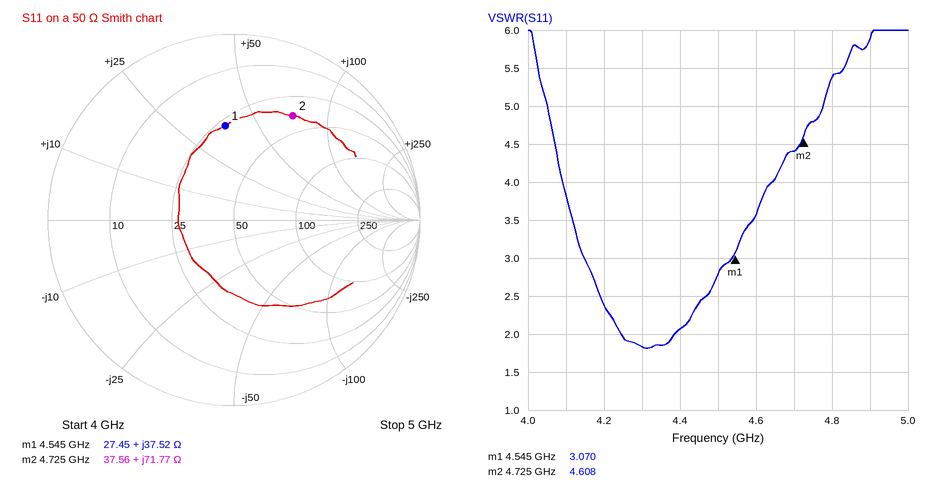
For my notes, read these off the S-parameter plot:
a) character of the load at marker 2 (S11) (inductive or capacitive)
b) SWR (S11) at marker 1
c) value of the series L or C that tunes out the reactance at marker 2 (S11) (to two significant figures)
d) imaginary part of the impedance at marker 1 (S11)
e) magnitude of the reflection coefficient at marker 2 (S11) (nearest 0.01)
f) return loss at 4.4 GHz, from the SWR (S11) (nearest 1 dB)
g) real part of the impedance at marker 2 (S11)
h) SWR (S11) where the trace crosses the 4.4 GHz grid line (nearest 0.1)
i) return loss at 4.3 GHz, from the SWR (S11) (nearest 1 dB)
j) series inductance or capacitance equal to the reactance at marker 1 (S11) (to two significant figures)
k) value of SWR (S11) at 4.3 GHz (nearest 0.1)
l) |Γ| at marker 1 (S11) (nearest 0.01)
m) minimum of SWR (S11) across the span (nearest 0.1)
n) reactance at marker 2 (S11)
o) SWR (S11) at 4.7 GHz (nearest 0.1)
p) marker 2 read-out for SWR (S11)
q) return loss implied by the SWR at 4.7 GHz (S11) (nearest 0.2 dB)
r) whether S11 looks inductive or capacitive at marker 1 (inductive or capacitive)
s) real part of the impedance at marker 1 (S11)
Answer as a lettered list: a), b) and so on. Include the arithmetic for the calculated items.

a) inductive
b) 3.070
c) C = 1/(2π × 4.725 GHz × 71.77 Ω) ≈ 469 fF, so 470 fF to two significant figures
d) +37.52 Ω
e) 0.64
f) −20 log10((2.1 − 1)/(2.1 + 1)) ≈ 9 dB
g) 37.56 Ω
h) 2.1
i) −20 log10((1.8 − 1)/(1.8 + 1)) ≈ 11 dB
j) L = 37.52 Ω/(2π × 4.545 GHz) ≈ 1.3 nH
k) 1.8
l) 0.51
m) 1.8
n) +71.77 Ω
o) 4.4
p) 4.608
q) −20 log10((4.4 − 1)/(4.4 + 1)) ≈ 4.0 dB
r) inductive
s) 27.45 Ω
